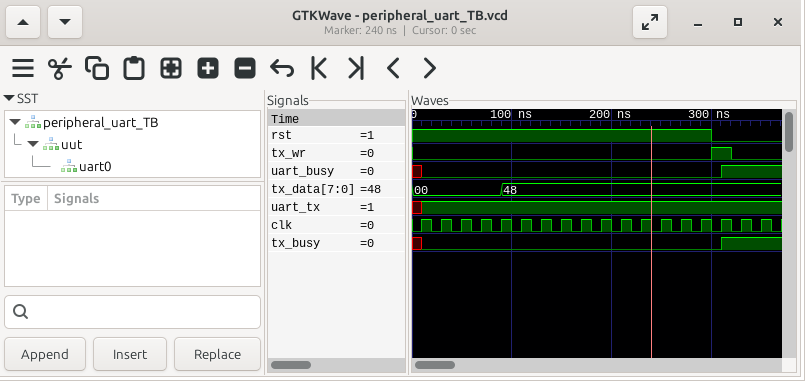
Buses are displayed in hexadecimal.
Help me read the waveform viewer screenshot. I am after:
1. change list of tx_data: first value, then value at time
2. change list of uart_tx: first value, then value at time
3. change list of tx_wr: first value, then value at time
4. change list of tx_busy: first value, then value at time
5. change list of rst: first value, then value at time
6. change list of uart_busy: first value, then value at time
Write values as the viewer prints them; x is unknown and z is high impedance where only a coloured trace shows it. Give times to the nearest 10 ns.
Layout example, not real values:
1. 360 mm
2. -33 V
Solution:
1. 00, 48 at 90 ns
2. x, 1 at 10 ns
3. 0, 1 at 300 ns, 0 at 320 ns
4. x, 0 at 10 ns, 1 at 310 ns
5. 1, 0 at 300 ns
6. x, 0 at 10 ns, 1 at 310 ns
